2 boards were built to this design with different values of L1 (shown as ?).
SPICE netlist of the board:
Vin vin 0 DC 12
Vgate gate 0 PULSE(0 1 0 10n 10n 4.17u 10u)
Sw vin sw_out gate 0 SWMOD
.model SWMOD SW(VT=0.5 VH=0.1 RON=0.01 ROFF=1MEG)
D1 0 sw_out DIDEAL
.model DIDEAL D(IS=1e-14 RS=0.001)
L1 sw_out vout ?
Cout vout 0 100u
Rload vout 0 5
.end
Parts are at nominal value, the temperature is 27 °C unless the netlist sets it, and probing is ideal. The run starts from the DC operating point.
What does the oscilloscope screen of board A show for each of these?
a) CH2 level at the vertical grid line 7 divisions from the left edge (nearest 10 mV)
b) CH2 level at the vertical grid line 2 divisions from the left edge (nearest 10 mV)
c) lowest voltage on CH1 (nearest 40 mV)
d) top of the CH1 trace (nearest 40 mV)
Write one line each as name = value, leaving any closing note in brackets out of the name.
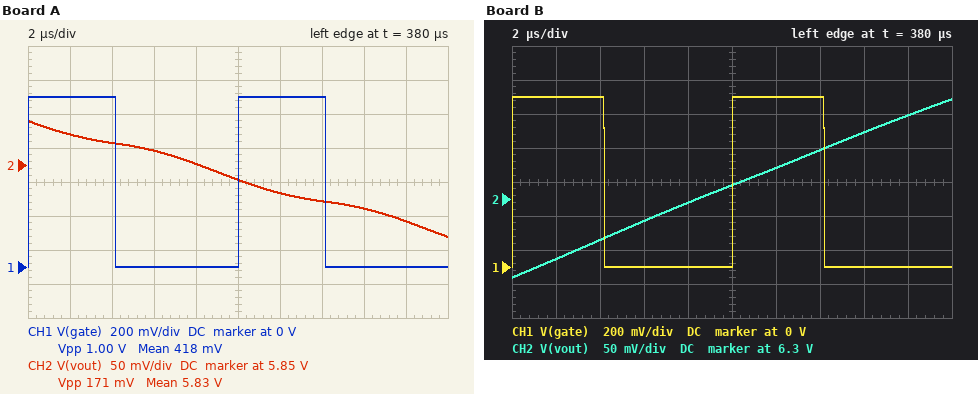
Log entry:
CH2 level at the vertical grid line 7 divisions from the left edge = 5.80 V
CH2 level at the vertical grid line 2 divisions from the left edge = 5.88 V
lowest voltage on CH1 = 0 V
top of the CH1 trace = 1.00 V
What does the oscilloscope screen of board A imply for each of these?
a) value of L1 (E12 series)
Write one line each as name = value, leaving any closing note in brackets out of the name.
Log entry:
value of L1 = 33 µH
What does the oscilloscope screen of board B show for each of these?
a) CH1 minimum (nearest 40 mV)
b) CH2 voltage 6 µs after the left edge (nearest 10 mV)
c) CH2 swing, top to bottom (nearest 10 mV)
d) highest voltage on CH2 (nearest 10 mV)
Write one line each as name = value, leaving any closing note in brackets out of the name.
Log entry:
CH1 minimum = 0 V
CH2 voltage 6 µs after the left edge = 6.27 V
CH2 swing, top to bottom = 260 mV
highest voltage on CH2 = 6.45 V
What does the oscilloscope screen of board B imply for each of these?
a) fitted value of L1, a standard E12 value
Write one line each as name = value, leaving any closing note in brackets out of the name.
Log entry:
fitted value of L1, a standard E12 value = 270 µH
